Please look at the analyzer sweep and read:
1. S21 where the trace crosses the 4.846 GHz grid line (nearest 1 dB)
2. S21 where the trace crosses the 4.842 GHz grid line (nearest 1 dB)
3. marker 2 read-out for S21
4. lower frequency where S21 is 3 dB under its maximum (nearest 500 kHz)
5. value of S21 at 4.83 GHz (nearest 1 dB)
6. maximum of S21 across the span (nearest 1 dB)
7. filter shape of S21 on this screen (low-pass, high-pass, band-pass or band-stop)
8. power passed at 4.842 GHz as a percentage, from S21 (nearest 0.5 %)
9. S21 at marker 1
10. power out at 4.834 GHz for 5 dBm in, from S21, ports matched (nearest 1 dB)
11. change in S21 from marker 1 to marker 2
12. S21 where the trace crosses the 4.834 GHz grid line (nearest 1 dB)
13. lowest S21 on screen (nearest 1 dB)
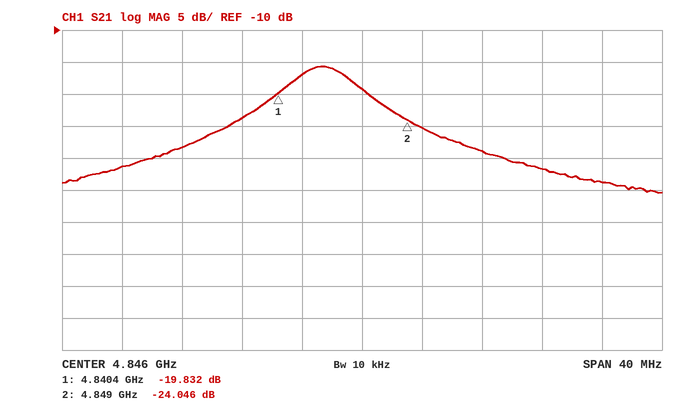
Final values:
-19 dB
-17 dB
-24.046 dB
4.8410 GHz
-31 dB
-16 dB
band-pass
2.0 %
-19.832 dB
-23 dBm
-4.214 dB
-28 dB
-35 dB
